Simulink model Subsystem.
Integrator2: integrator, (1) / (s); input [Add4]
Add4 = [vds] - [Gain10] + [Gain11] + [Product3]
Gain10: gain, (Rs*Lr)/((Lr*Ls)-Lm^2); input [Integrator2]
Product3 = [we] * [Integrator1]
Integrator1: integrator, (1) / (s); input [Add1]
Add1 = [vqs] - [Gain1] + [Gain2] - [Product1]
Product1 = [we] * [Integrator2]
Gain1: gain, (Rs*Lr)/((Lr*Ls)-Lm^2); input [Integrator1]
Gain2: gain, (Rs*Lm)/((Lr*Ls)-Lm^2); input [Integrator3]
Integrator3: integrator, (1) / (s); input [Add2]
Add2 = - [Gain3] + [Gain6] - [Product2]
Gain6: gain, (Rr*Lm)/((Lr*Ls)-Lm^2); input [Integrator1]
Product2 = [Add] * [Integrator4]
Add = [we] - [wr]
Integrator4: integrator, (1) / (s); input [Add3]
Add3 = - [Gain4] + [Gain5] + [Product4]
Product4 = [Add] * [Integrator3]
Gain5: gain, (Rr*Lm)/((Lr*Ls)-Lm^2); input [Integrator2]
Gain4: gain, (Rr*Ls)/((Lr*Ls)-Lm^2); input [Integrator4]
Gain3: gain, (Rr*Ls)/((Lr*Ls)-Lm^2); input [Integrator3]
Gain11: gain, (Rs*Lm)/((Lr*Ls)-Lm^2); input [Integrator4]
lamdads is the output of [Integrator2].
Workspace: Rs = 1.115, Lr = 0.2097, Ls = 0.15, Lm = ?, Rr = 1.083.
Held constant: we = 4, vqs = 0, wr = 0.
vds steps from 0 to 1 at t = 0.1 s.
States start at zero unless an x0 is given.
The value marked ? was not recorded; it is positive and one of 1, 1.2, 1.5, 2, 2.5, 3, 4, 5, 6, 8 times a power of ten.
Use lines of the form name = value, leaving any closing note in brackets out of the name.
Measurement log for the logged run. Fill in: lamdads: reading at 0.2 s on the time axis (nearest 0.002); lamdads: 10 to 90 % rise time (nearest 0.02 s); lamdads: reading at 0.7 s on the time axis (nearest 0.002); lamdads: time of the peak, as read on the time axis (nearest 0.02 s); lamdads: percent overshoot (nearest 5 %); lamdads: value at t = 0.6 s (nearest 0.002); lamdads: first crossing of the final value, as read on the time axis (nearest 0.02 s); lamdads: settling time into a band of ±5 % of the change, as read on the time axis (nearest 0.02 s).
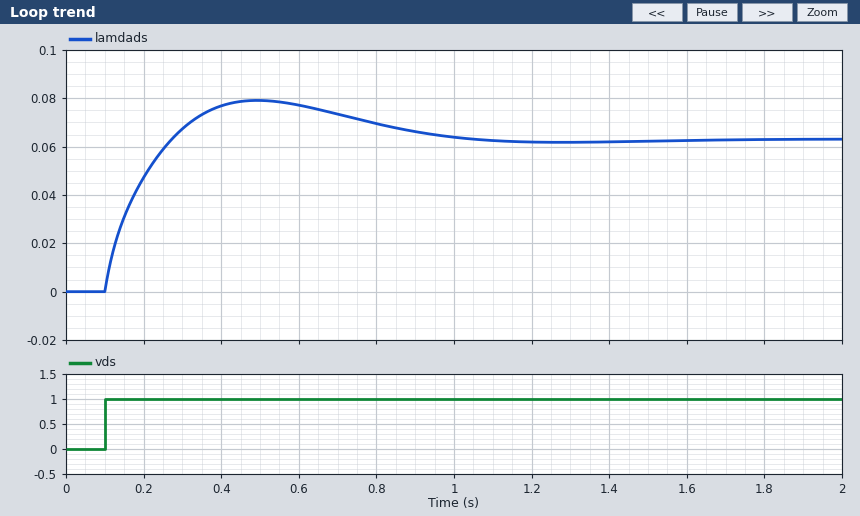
lamdads: reading at 0.2 s on the time axis = 0.048
lamdads: 10 to 90 % rise time = 0.14 s
lamdads: reading at 0.7 s on the time axis = 0.074
lamdads: time of the peak, as read on the time axis = 0.50 s
lamdads: percent overshoot = 25 %
lamdads: value at t = 0.6 s = 0.078
lamdads: first crossing of the final value, as read on the time axis = 0.28 s
lamdads: settling time into a band of ±5 % of the change, as read on the time axis = 0.90 s
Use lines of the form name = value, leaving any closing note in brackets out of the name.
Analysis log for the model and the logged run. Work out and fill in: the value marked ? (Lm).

the value marked ? = 0.15
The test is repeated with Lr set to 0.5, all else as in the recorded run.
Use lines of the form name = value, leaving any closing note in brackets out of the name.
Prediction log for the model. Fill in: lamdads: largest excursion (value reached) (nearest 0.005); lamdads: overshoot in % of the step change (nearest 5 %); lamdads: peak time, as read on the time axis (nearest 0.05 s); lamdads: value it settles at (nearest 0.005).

lamdads: largest excursion (value reached) = 0.090
lamdads: overshoot in % of the step change = 15 %
lamdads: peak time, as read on the time axis = 0.50 s
lamdads: value it settles at = 0.080
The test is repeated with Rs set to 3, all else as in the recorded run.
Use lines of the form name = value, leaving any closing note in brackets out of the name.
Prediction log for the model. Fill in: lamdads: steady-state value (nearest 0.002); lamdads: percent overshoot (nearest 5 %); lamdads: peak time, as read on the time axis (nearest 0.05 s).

lamdads: steady-state value = 0.032
lamdads: percent overshoot = 10 %
lamdads: peak time, as read on the time axis = 0.50 s
